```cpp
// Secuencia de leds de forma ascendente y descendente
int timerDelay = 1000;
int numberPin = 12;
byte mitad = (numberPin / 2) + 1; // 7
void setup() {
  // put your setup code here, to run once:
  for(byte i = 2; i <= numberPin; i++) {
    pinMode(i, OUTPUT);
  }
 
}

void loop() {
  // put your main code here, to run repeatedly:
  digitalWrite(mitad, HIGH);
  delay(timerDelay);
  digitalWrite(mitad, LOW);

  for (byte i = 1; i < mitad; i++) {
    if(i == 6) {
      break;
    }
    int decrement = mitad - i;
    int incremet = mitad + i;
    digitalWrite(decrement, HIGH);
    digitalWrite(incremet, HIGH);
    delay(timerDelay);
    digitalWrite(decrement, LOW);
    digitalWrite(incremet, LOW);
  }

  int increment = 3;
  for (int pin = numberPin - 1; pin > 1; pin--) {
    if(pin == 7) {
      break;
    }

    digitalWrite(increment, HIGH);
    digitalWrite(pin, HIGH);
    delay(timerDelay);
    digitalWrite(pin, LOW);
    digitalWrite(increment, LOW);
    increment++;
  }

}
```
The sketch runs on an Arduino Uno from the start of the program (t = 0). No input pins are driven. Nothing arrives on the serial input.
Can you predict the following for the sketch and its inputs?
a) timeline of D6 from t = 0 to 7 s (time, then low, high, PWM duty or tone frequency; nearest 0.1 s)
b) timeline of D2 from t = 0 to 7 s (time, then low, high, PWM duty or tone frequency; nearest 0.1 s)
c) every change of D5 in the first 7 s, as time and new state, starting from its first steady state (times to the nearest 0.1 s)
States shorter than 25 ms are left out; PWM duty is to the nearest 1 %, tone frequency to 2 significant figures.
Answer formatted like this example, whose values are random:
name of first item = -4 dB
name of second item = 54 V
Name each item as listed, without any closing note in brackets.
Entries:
timeline of D6 from t = 0 to 7 s = 0 s low; 1 s high; 2 s low
timeline of D2 from t = 0 to 7 s = 0 s low; 5 s high; 6 s low
every change of D5 in the first 7 s, as time and new state, starting from its first steady state = 0 s low; 2 s high; 3 s low
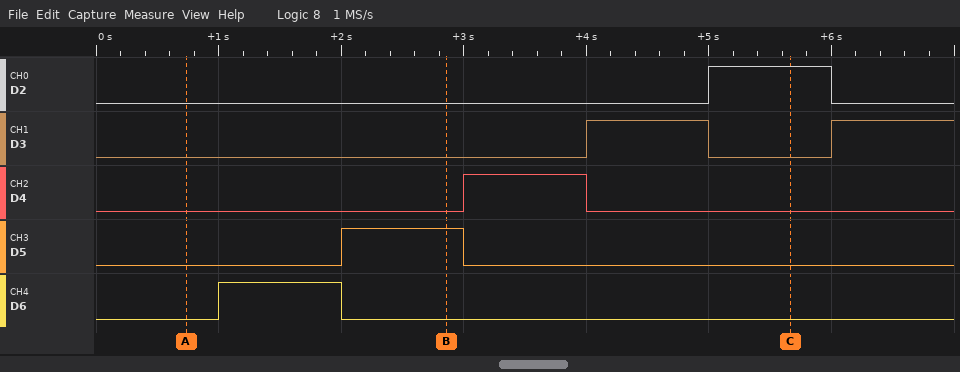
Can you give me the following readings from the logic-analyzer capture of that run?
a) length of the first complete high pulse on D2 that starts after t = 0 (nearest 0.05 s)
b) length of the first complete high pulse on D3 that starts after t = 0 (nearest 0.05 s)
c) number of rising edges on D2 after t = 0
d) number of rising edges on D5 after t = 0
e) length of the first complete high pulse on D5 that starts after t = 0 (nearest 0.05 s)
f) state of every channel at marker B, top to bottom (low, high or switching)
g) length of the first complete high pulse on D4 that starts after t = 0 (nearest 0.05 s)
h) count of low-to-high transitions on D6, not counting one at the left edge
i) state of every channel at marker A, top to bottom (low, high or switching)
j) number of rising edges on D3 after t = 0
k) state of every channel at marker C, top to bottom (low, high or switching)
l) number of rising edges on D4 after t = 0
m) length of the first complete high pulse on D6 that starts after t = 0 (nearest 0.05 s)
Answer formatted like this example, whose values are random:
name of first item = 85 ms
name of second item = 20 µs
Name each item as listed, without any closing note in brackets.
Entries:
length of the first complete high pulse on D2 that starts after t = 0 = 1.00 s
length of the first complete high pulse on D3 that starts after t = 0 = 1.00 s
number of rising edges on D2 after t = 0 = 1
number of rising edges on D5 after t = 0 = 1
length of the first complete high pulse on D5 that starts after t = 0 = 1.00 s
state of every channel at marker B, top to bottom = D2 low, D3 low, D4 low, D5 high, D6 low
length of the first complete high pulse on D4 that starts after t = 0 = 1.00 s
count of low-to-high transitions on D6, not counting one at the left edge = 1
state of every channel at marker A, top to bottom = D2 low, D3 low, D4 low, D5 low, D6 low
number of rising edges on D3 after t = 0 = 2
state of every channel at marker C, top to bottom = D2 high, D3 low, D4 low, D5 low, D6 low
number of rising edges on D4 after t = 0 = 1
length of the first complete high pulse on D6 that starts after t = 0 = 1.00 s
